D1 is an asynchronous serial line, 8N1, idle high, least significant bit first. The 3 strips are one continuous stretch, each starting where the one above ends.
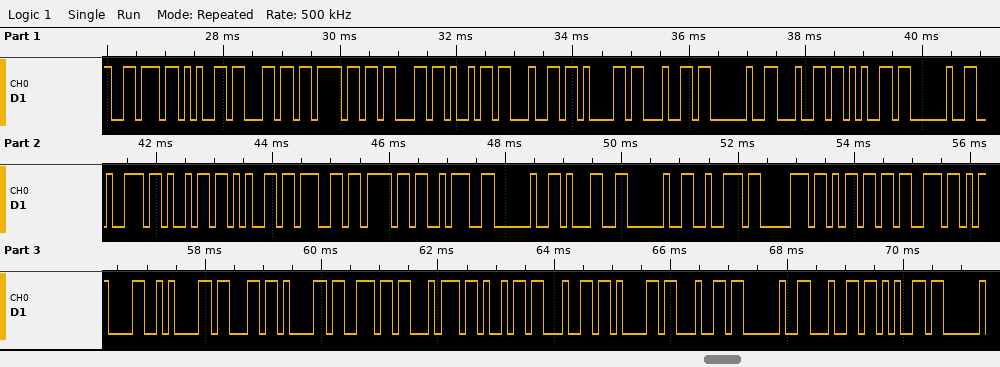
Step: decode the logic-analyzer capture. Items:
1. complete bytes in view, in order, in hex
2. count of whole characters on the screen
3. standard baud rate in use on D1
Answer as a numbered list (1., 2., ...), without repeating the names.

1. 76 65 6C 6F 63 69 64 61 64 20 64 65 20 72 69 65 67 6F 3A 20 31 20 72 70 6D 73 0D 0A 63 61 6E 74 69 64 61 64 20 64 65
2. 39
3. 9600 baud
